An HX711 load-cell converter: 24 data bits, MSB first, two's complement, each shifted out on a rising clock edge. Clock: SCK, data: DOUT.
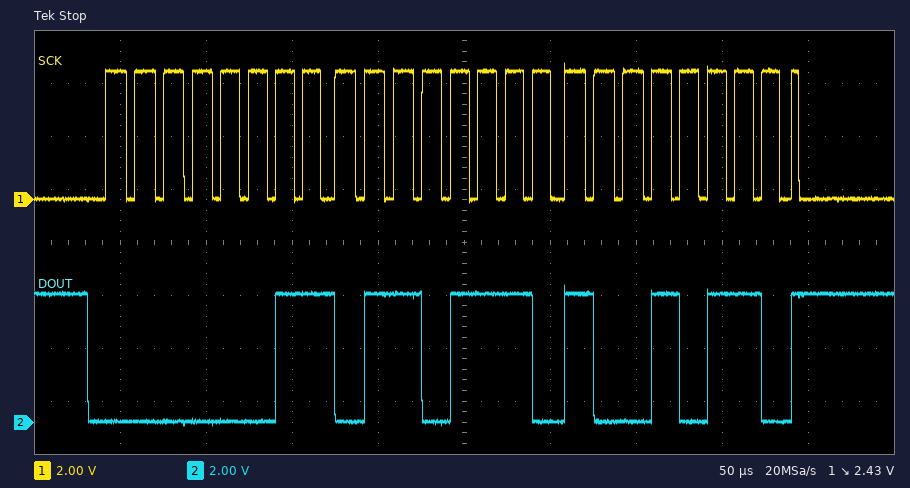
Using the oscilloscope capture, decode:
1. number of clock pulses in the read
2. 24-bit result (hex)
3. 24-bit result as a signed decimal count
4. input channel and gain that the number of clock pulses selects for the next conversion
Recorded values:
25
0x036E96
224918
channel A, gain 128
